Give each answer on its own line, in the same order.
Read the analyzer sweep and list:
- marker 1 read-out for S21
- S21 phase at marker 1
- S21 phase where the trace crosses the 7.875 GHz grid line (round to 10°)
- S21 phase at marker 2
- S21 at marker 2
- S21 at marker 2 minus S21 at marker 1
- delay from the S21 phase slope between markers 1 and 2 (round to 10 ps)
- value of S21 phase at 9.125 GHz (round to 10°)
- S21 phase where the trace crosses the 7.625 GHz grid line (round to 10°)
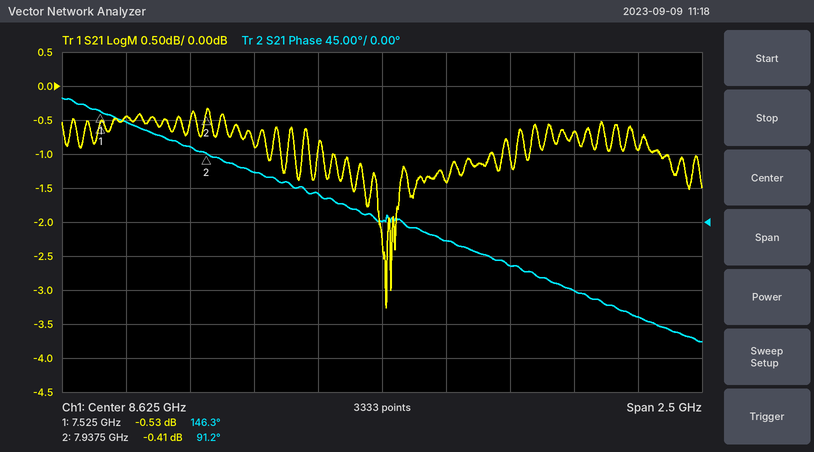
-0.53 dB
146.3°
100°
91.2°
-0.41 dB
0.12 dB
370 ps
-60°
130°
